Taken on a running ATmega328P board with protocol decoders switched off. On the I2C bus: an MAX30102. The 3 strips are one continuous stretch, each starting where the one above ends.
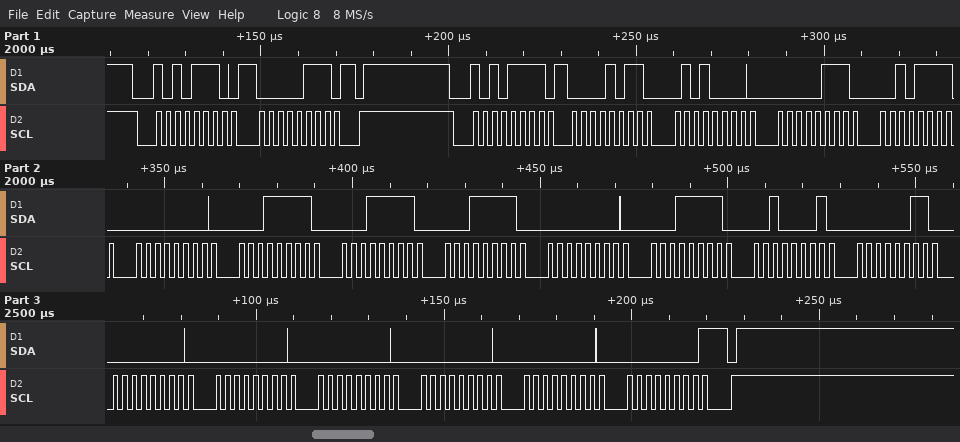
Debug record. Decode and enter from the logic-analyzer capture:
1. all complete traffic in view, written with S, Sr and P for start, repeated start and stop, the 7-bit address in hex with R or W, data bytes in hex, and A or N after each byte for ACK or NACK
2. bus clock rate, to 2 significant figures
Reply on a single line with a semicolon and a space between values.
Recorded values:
S 57W A 07 A P S 57R A 0B A 50 A 07 A 2F A 00 A 1F A 1F A 1F A 00 A 1F A 21 A 03 A 00 A 00 A 00 A 00 A 00 A 00 N P; 400 kHz
